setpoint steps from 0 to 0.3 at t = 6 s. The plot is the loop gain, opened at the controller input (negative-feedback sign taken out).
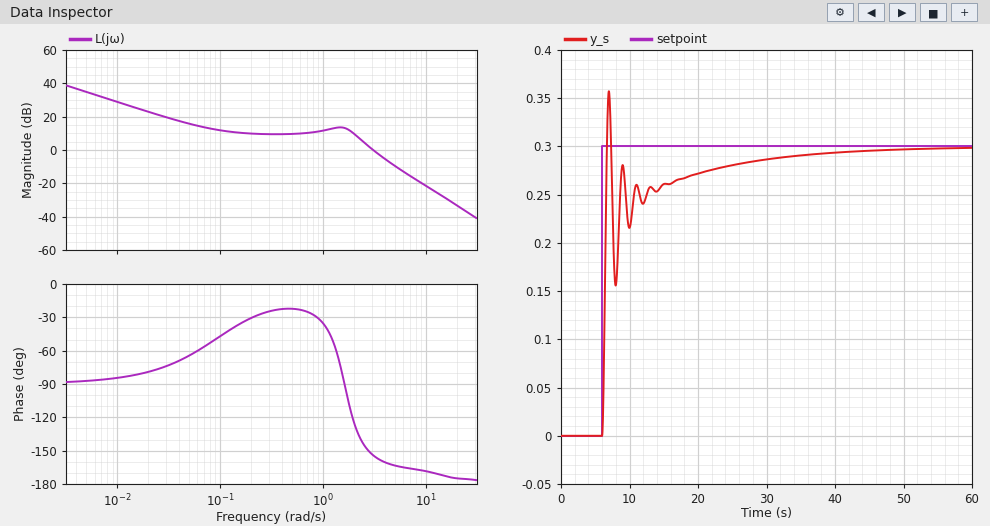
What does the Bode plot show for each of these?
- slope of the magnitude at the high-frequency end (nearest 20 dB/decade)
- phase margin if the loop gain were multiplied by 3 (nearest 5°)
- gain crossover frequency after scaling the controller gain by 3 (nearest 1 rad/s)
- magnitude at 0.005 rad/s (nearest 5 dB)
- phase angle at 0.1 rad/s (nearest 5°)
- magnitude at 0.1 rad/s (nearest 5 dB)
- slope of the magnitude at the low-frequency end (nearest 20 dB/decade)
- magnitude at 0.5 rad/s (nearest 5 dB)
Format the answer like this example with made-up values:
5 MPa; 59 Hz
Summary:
-40 dB/decade; 15°; 5 rad/s; 35 dB; -45°; 10 dB; -20 dB/decade; 10 dB
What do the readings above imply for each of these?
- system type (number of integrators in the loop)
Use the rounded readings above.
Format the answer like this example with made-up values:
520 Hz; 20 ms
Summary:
1
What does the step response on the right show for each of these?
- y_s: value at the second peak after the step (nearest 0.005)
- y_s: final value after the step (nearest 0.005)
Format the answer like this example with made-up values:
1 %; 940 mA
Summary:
0.280; 0.300
